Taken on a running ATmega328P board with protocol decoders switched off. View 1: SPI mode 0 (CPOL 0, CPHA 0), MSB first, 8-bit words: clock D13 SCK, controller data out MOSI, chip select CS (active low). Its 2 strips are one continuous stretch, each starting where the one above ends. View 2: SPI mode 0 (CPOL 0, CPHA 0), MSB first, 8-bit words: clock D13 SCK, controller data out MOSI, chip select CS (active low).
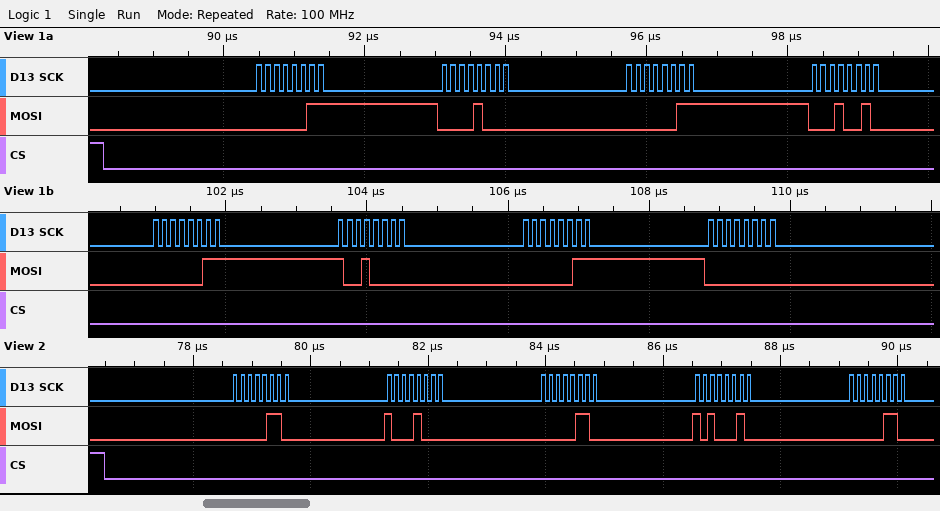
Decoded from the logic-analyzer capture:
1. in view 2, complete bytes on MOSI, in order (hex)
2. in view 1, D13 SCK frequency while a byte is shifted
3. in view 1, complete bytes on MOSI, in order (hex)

0x06 0x88 0x06 0xA2 0x06
8 MHz
03 08 03 12 03 90 03 00
